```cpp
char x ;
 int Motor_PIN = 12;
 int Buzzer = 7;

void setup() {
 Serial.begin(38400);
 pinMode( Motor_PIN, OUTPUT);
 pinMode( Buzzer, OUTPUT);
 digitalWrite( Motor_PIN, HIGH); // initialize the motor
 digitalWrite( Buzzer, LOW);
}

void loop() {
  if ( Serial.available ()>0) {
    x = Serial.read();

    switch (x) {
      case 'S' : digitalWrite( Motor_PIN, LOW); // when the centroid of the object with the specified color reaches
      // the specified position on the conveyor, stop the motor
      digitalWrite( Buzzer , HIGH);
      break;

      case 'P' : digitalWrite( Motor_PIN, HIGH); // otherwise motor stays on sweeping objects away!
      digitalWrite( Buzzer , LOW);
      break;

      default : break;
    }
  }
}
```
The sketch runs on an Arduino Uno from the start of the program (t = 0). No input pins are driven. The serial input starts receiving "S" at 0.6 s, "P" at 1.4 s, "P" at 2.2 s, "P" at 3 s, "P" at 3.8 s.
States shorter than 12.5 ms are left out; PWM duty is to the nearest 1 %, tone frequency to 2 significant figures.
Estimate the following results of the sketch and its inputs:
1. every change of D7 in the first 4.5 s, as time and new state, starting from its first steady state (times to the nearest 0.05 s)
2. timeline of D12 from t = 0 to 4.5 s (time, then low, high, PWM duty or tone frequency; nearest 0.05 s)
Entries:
0 s low; 0.6 s high; 1.4 s low
0 s high; 0.6 s low; 1.4 s high
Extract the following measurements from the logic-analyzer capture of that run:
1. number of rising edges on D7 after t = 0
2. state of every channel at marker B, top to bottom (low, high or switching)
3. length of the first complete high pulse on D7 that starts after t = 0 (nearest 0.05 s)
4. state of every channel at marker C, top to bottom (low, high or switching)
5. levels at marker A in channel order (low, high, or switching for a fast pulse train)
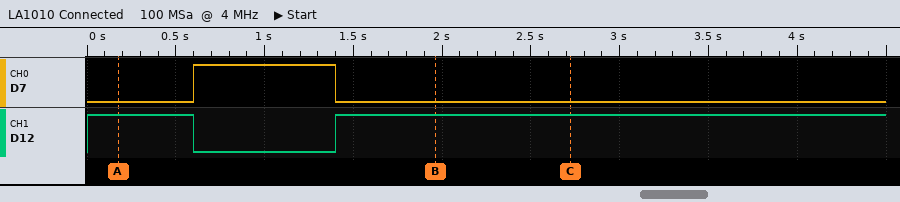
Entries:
1
D7 low, D12 high
0.80 s
D7 low, D12 high
D7 low, D12 high
